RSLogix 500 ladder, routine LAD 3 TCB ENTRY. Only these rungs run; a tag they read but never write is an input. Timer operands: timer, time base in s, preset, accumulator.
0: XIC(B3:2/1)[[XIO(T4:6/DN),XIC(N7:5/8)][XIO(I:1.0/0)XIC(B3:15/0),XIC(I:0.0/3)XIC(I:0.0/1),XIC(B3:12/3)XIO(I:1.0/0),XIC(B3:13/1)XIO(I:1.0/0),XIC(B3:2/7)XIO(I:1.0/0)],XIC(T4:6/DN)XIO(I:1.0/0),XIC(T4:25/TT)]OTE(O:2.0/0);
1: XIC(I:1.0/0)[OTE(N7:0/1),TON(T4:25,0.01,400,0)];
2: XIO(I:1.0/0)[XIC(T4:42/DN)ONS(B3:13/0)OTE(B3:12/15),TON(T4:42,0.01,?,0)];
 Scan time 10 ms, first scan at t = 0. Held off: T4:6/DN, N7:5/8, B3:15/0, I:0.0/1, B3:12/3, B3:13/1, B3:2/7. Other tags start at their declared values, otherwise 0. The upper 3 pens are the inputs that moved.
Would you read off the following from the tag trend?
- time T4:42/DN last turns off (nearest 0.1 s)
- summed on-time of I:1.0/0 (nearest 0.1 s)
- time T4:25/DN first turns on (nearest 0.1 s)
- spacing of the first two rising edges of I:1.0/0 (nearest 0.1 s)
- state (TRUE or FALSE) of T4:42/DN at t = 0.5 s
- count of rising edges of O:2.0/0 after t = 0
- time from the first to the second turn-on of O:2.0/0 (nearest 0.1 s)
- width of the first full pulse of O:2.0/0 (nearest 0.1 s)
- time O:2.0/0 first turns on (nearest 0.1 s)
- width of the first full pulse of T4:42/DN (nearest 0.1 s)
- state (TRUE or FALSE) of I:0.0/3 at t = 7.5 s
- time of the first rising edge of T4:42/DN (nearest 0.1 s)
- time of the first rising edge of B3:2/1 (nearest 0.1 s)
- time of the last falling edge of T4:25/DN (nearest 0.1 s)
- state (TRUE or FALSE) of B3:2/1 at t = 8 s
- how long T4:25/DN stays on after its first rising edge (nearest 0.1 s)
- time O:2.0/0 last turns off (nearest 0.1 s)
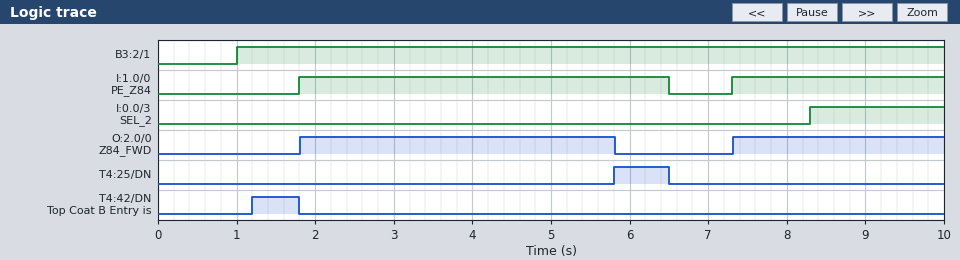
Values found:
1.8 s
7.4 s
5.8 s
5.5 s
FALSE
2
5.5 s
4.0 s
1.8 s
0.6 s
FALSE
1.2 s
1.0 s
6.5 s
TRUE
0.7 s
5.8 s
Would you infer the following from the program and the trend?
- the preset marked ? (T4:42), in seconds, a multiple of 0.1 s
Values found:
1.2 s
